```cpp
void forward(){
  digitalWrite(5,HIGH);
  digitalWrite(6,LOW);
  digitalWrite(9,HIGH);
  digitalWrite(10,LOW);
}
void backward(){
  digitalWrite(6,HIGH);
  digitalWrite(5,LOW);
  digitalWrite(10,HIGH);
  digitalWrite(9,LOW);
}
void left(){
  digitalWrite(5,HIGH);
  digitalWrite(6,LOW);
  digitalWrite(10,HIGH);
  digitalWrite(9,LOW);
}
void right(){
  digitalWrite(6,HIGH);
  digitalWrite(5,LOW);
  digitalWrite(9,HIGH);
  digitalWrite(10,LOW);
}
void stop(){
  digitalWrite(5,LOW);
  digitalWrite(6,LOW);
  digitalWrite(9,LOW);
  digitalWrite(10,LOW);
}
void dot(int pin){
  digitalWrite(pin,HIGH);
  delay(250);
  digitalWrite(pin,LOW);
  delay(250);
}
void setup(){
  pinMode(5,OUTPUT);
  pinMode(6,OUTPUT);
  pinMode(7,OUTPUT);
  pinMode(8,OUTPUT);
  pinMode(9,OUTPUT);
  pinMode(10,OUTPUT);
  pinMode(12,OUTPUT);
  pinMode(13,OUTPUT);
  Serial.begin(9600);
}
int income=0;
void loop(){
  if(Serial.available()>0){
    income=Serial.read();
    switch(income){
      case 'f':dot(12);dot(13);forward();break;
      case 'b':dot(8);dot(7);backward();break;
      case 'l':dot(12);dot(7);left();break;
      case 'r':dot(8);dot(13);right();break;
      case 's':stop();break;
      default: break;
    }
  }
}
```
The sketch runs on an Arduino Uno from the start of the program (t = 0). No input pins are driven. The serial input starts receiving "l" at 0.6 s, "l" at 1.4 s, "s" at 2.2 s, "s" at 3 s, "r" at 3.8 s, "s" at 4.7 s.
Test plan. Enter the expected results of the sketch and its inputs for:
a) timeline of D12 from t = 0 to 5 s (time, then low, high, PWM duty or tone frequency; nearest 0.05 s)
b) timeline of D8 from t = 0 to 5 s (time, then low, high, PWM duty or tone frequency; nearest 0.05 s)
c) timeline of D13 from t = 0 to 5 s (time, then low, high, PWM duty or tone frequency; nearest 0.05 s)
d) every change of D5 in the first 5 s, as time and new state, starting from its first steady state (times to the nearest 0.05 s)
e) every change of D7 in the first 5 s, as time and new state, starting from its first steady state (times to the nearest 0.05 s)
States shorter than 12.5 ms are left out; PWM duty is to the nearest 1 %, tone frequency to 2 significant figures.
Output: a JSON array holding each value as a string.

["0 s low; 0.6 s high; 0.85 s low; 1.6 s high; 1.85 s low", "0 s low; 3.8 s high; 4.05 s low", "0 s low; 4.3 s high; 4.55 s low", "0 s low; 1.6 s high; 2.6 s low", "0 s low; 1.1 s high; 1.35 s low; 2.1 s high; 2.35 s low"]
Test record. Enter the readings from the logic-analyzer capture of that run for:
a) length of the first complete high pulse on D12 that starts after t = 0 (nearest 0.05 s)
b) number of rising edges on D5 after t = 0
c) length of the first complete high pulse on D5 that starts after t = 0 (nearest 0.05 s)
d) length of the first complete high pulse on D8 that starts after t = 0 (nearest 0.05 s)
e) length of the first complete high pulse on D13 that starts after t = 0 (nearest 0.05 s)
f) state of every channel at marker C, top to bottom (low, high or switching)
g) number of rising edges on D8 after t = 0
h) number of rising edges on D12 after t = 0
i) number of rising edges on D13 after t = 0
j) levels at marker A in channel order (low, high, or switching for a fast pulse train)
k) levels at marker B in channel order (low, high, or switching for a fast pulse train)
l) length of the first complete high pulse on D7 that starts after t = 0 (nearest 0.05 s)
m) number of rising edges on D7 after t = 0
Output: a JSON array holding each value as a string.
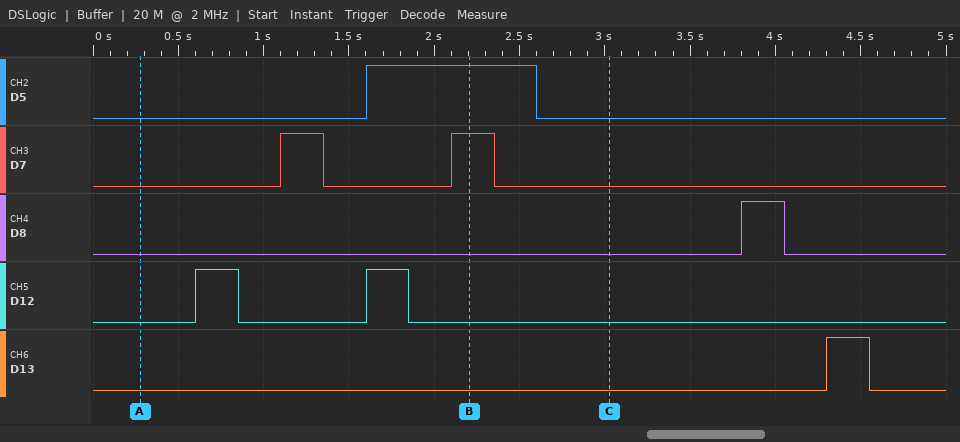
["0.25 s", "1", "1.00 s", "0.25 s", "0.25 s", "D5 low, D7 low, D8 low, D12 low, D13 low", "1", "2", "1", "D5 low, D7 low, D8 low, D12 low, D13 low", "D5 high, D7 high, D8 low, D12 low, D13 low", "0.25 s", "2"]
